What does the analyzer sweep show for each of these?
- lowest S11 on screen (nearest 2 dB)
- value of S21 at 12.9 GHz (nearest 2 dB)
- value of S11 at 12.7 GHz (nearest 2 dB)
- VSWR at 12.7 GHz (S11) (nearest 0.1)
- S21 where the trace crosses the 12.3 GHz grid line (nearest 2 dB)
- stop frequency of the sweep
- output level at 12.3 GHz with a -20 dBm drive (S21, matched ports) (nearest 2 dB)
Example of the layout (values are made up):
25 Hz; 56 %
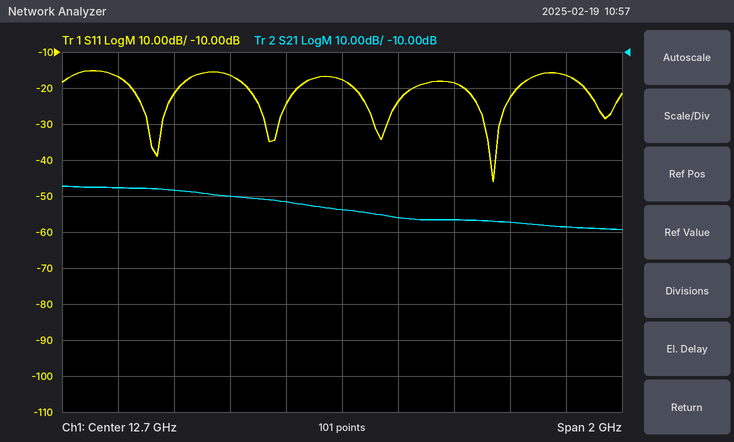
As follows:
-46 dB; -56 dB; -18 dB; 1.3; -50 dB; 13.7 GHz; -70 dBm
